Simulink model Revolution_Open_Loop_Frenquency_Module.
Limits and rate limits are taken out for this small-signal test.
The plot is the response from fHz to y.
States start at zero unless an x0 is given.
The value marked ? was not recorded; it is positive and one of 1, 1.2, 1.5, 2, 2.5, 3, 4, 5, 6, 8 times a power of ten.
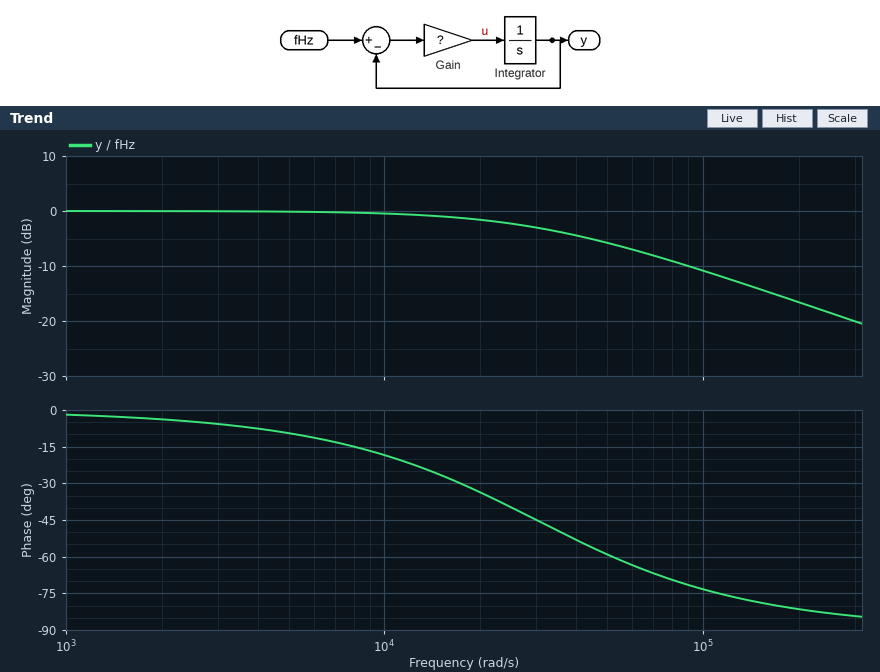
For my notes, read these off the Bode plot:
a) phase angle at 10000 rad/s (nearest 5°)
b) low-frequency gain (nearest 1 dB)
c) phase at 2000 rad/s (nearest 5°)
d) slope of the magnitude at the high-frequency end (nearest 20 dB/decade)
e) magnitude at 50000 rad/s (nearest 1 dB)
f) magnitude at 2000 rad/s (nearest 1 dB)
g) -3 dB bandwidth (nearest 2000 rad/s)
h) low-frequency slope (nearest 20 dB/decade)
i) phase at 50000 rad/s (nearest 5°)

-20°
0 dB
-5°
-20 dB/decade
-6 dB
0 dB
30000 rad/s
0 dB/decade
-60°
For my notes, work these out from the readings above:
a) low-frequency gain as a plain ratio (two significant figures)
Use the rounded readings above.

1.0
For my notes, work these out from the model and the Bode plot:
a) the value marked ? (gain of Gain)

30000
